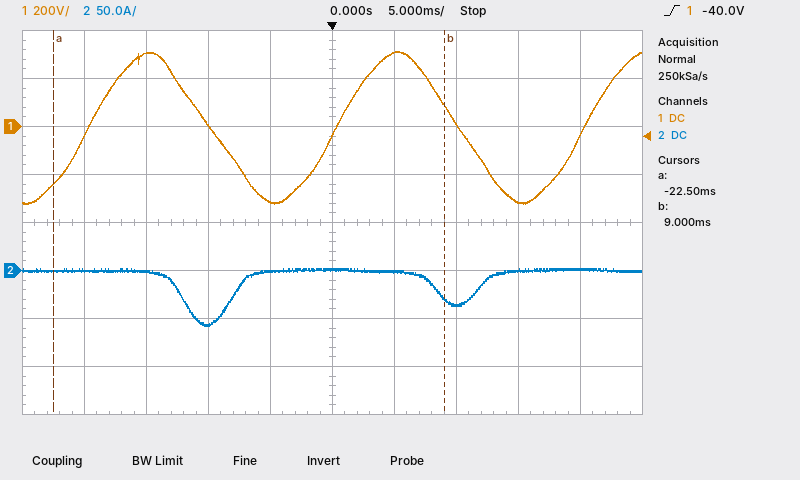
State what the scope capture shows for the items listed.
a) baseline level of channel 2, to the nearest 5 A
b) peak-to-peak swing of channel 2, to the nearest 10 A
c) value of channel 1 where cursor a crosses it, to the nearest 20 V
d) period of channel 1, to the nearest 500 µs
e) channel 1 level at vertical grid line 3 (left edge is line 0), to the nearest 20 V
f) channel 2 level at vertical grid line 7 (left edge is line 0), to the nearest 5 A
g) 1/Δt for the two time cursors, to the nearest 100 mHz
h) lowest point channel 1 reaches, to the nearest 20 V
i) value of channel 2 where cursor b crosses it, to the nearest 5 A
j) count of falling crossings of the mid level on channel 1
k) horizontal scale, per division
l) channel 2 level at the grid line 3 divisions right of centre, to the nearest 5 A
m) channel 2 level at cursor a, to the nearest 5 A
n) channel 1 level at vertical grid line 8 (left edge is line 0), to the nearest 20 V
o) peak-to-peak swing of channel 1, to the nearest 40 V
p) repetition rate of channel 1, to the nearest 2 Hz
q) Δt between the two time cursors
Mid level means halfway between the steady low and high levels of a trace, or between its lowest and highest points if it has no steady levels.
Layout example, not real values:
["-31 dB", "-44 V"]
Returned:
["0 A", "60 A", "-240 V", "20.0 ms", "0 V", "-35 A", "31.7 Hz", "-320 V", "-30 A", "2", "5 ms", "0 A", "0 A", "-320 V", "640 V", "50 Hz", "31.5 ms"]
